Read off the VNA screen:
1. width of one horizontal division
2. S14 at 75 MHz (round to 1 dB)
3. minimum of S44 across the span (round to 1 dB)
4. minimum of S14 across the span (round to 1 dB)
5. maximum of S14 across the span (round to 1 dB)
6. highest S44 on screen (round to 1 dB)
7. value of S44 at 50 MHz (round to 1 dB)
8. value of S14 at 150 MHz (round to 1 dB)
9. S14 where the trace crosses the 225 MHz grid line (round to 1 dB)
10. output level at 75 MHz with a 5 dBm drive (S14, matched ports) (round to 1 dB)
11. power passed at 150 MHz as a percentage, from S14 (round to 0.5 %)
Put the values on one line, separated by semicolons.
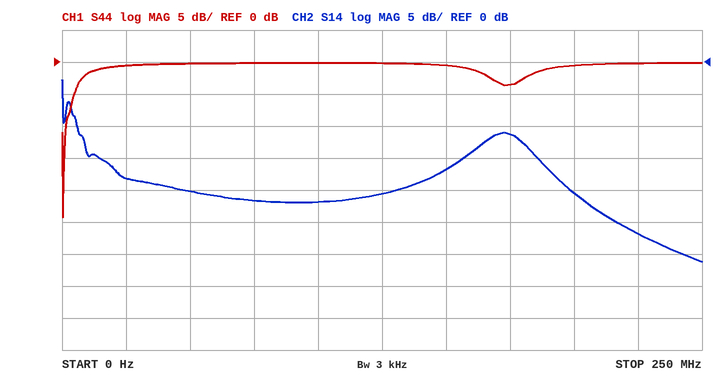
25 MHz; -22 dB; -24 dB; -31 dB; -3 dB; 0 dB; 0 dB; -17 dB; -27 dB; -17 dBm; 2.0 %
